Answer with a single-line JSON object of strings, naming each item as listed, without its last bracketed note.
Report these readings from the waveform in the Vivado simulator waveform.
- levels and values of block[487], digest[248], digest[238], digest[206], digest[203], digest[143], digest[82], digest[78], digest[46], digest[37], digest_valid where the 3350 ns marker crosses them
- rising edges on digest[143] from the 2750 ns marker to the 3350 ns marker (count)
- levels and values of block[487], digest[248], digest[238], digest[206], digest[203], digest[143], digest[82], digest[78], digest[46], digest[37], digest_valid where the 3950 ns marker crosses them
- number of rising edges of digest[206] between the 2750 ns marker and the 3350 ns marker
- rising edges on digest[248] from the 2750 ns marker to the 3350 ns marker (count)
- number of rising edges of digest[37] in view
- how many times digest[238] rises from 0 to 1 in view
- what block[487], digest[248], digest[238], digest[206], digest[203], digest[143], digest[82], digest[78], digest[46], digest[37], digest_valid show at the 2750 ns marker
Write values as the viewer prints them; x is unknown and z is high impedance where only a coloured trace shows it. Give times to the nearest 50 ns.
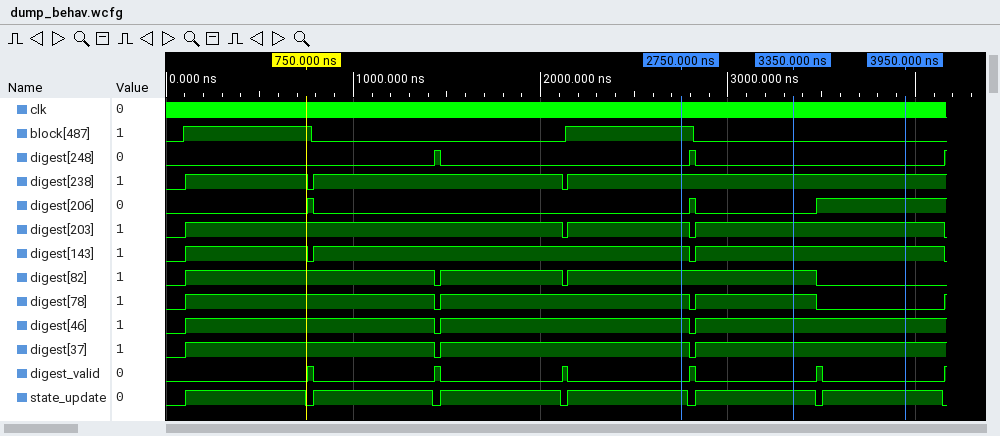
{"levels and values of block[487], digest[248], digest[238], digest[206], digest[203], digest[143], digest[82], digest[78], digest[46], digest[37], digest_valid where the 3350 ns marker crosses them": "block[487]=0, digest[248]=0, digest[238]=1, digest[206]=0, digest[203]=1, digest[143]=1, digest[82]=1, digest[78]=1, digest[46]=1, digest[37]=1, digest_valid=0", "rising edges on digest[143] from the 2750 ns marker to the 3350 ns marker": "1", "levels and values of block[487], digest[248], digest[238], digest[206], digest[203], digest[143], digest[82], digest[78], digest[46], digest[37], digest_valid where the 3950 ns marker crosses them": "block[487]=0, digest[248]=0, digest[238]=1, digest[206]=1, digest[203]=1, digest[143]=1, digest[82]=0, digest[78]=0, digest[46]=1, digest[37]=1, digest_valid=0", "number of rising edges of digest[206] between the 2750 ns marker and the 3350 ns marker": "1", "rising edges on digest[248] from the 2750 ns marker to the 3350 ns marker": "1", "number of rising edges of digest[37] in view": "3", "how many times digest[238] rises from 0 to 1 in view": "3", "what block[487], digest[248], digest[238], digest[206], digest[203], digest[143], digest[82], digest[78], digest[46], digest[37], digest_valid show at the 2750 ns marker": "block[487]=1, digest[248]=0, digest[238]=1, digest[206]=0, digest[203]=1, digest[143]=1, digest[82]=1, digest[78]=1, digest[46]=1, digest[37]=1, digest_valid=0"}
